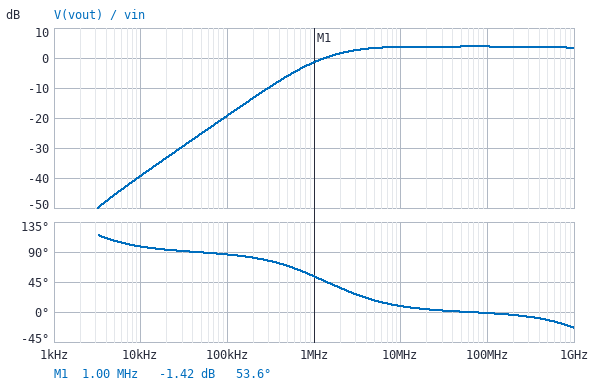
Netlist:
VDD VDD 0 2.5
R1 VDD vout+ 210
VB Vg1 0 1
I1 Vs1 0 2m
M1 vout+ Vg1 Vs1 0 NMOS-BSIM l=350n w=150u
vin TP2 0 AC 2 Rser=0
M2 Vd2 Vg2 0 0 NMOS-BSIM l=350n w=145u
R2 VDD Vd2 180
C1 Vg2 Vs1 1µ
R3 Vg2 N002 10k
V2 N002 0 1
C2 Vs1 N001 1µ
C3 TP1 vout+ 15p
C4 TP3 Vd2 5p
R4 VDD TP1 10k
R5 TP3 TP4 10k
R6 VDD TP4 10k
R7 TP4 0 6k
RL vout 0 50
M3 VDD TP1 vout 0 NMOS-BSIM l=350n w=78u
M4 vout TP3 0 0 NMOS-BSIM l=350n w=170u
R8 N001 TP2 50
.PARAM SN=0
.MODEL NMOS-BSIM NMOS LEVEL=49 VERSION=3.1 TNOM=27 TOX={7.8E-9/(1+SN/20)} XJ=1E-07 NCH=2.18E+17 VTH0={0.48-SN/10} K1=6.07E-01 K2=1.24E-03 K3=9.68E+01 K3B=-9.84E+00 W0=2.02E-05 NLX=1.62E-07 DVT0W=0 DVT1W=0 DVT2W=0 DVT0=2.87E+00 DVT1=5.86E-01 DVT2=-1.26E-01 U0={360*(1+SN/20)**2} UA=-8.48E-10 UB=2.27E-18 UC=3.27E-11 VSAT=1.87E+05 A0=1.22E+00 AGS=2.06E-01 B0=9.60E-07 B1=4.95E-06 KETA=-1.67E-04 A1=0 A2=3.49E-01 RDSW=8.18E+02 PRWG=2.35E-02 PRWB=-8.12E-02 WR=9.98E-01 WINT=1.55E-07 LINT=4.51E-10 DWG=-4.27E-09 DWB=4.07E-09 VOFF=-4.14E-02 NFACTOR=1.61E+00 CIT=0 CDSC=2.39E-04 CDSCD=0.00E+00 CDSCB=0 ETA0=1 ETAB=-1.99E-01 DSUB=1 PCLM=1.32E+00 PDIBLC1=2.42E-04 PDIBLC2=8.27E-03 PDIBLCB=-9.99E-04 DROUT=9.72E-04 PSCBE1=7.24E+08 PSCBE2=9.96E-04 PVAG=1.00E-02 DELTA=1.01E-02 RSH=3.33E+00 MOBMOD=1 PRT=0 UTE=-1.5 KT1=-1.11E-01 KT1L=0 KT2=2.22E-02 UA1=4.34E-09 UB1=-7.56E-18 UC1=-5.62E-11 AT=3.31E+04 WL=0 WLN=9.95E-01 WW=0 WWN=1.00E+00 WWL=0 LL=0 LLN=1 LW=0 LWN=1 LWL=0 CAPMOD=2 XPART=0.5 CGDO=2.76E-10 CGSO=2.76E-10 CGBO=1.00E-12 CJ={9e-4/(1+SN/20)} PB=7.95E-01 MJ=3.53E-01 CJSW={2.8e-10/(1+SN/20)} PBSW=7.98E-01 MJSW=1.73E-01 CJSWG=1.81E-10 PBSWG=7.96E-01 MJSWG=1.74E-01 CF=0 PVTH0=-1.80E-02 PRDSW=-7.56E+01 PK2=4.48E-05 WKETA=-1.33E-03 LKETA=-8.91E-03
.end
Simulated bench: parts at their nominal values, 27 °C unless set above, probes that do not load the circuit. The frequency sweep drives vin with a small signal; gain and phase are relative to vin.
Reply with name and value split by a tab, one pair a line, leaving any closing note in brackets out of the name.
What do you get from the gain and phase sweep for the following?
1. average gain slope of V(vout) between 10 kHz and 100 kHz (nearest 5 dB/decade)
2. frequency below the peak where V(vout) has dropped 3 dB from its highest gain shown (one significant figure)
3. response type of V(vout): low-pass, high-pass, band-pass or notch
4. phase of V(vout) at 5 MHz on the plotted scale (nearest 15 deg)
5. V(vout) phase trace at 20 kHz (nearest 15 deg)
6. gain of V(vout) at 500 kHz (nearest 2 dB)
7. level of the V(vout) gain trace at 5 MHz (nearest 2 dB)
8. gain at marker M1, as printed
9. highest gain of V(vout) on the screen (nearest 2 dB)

average gain slope of V(vout) between 10 kHz and 100 kHz	20 dB/decade
frequency below the peak where V(vout) has dropped 3 dB from its highest gain shown	2 MHz
response type of V(vout): low-pass, high-pass, band-pass or notch	high-pass
phase of V(vout) at 5 MHz on the plotted scale	15 deg
V(vout) phase trace at 20 kHz	90 deg
gain of V(vout) at 500 kHz	-6 dB
level of the V(vout) gain trace at 5 MHz	4 dB
gain at marker M1, as printed	-1.42 dB
highest gain of V(vout) on the screen	4 dB
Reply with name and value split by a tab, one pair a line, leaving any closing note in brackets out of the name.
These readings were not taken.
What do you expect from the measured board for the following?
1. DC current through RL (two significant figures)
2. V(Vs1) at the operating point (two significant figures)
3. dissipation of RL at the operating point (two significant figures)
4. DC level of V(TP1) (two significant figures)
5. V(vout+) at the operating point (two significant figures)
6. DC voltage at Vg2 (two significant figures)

DC current through RL	11 mA
V(Vs1) at the operating point	170 mV
dissipation of RL at the operating point	5.6 mW
DC level of V(TP1)	2.5 V
V(vout+) at the operating point	2.1 V
DC voltage at Vg2	1.0 V
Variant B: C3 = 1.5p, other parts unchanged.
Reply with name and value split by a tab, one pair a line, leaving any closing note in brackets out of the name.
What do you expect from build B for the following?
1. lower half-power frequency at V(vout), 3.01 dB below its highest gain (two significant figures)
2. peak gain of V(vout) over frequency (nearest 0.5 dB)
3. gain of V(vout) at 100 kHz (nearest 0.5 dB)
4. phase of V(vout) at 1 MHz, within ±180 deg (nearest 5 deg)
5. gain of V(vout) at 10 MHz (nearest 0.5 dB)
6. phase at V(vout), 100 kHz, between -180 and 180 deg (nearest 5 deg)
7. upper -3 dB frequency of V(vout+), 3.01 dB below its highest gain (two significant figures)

lower half-power frequency at V(vout), 3.01 dB below its highest gain	6.0 MHz
peak gain of V(vout) over frequency	3.5 dB
gain of V(vout) at 100 kHz	-27.0 dB
phase of V(vout) at 1 MHz, within ±180 deg	70 deg
gain of V(vout) at 10 MHz	2.0 dB
phase at V(vout), 100 kHz, between -180 and 180 deg	90 deg
upper -3 dB frequency of V(vout+), 3.01 dB below its highest gain	5.2 GHz
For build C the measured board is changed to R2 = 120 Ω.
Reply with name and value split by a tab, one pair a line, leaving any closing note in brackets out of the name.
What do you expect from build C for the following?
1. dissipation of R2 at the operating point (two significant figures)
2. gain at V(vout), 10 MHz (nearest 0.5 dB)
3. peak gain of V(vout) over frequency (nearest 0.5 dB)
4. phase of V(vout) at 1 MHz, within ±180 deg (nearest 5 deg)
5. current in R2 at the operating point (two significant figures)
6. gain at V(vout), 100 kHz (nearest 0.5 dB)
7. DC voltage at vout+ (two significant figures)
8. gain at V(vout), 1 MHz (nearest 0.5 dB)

dissipation of R2 at the operating point	3.9 mW
gain at V(vout), 10 MHz	2.0 dB
peak gain of V(vout) over frequency	2.5 dB
phase of V(vout) at 1 MHz, within ±180 deg	50 deg
current in R2 at the operating point	5.7 mA
gain at V(vout), 100 kHz	-20.0 dB
DC voltage at vout+	2.1 V
gain at V(vout), 1 MHz	-2.5 dB
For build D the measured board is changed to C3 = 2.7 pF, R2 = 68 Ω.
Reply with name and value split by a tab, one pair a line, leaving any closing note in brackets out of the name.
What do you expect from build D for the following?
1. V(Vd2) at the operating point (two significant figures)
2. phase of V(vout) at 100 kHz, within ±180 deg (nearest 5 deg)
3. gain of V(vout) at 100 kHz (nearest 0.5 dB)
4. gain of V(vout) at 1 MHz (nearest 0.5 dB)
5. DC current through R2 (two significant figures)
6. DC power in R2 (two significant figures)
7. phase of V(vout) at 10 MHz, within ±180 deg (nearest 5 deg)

V(Vd2) at the operating point	2.1 V
phase of V(vout) at 100 kHz, within ±180 deg	90 deg
gain of V(vout) at 100 kHz	-31.0 dB
gain of V(vout) at 1 MHz	-11.5 dB
DC current through R2	5.8 mA
DC power in R2	2.3 mW
phase of V(vout) at 10 MHz, within ±180 deg	25 deg
